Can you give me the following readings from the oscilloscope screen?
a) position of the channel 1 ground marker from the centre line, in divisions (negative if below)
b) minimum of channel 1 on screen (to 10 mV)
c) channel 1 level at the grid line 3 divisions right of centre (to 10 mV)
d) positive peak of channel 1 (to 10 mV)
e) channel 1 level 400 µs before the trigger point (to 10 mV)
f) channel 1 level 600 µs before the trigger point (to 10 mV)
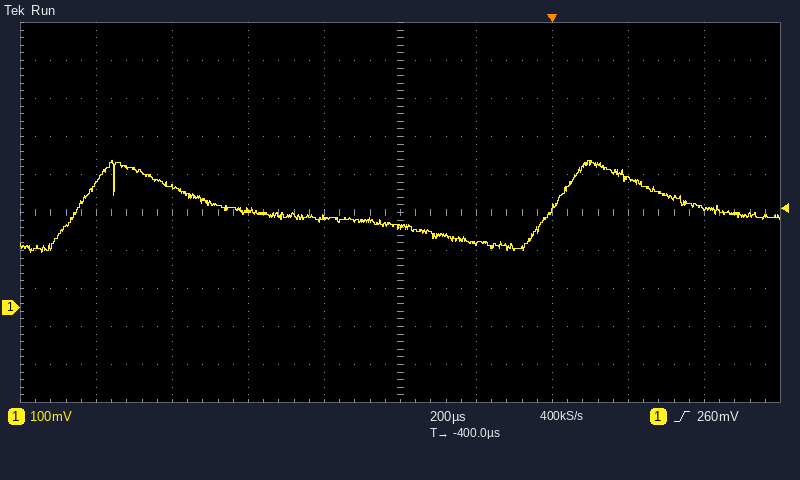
-2.5 div
140 mV
340 mV
390 mV
210 mV
240 mV
